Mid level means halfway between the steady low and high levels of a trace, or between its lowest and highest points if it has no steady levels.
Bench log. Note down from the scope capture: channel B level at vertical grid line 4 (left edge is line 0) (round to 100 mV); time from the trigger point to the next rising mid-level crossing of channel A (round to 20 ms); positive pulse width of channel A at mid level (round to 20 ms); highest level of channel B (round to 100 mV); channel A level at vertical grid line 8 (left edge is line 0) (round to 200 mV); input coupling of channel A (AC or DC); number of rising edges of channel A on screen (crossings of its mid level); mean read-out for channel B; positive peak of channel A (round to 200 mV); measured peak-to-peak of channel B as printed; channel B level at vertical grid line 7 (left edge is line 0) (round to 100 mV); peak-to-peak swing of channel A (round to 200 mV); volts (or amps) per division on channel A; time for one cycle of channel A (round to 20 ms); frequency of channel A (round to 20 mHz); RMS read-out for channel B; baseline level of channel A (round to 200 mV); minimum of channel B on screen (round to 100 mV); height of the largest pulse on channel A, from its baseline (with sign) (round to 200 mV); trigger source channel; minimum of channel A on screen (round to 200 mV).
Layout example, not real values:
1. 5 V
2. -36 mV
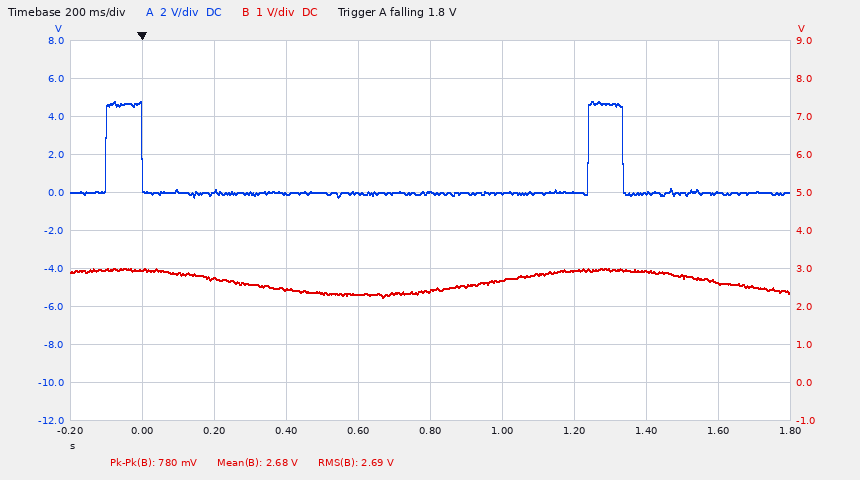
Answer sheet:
1. 2.3 V
2. 1.24 s
3. 100 ms
4. 3.0 V
5. 0.0 V
6. DC
7. 2
8. 2.68 V
9. 4.8 V
10. 780 mV
11. 2.9 V
12. 5.0 V
13. 2 V
14. 1.34 s
15. 740 mHz
16. 2.69 V
17. 0.0 V
18. 2.2 V
19. +4.8 V
20. channel A
21. -200 mV
